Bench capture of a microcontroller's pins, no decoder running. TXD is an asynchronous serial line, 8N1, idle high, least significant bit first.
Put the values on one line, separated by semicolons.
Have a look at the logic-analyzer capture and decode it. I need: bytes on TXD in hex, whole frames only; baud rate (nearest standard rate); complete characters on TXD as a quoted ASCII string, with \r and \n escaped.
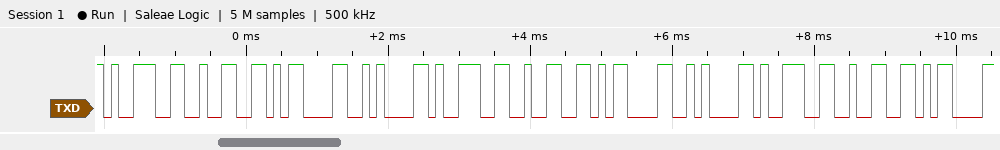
0x39 0x32 0x0D 0x0A 0x39 0x32 0x0D 0x0A 0x39 0x32 0x0D; 9600 baud; "92\r\n92\r\n92\r"
